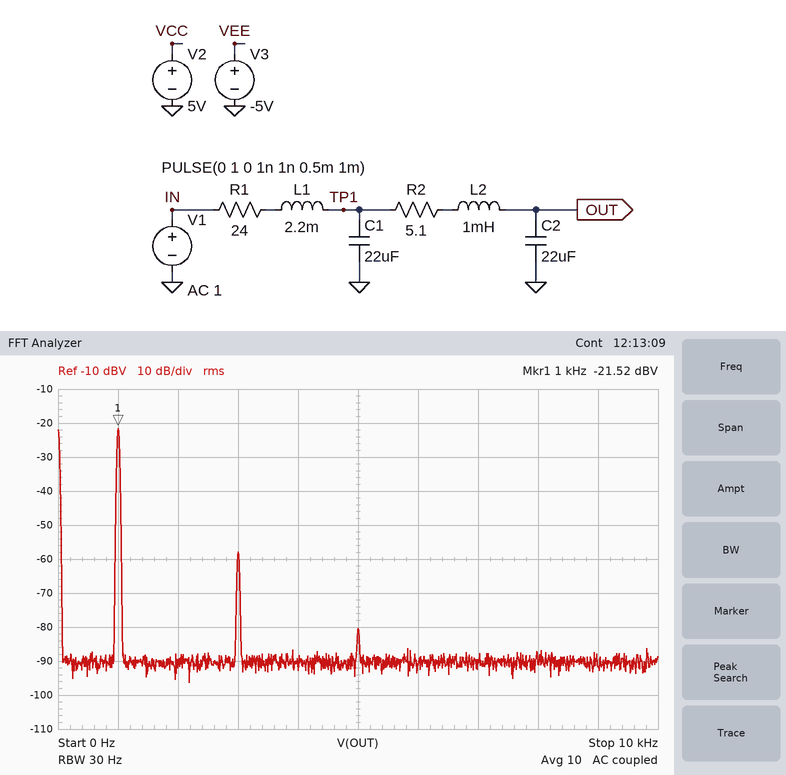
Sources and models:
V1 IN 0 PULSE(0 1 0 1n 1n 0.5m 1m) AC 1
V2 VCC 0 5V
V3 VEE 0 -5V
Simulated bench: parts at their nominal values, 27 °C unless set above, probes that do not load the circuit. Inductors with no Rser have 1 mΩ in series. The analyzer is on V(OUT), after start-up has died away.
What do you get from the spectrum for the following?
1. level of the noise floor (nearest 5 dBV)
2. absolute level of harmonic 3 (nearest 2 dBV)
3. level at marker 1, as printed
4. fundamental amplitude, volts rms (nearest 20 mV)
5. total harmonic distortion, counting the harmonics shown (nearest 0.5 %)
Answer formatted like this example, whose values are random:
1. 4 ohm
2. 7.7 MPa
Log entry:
1. -90 dBV
2. -58 dBV
3. -21.52 dBV
4. 80 mV
5. 1.5 %
